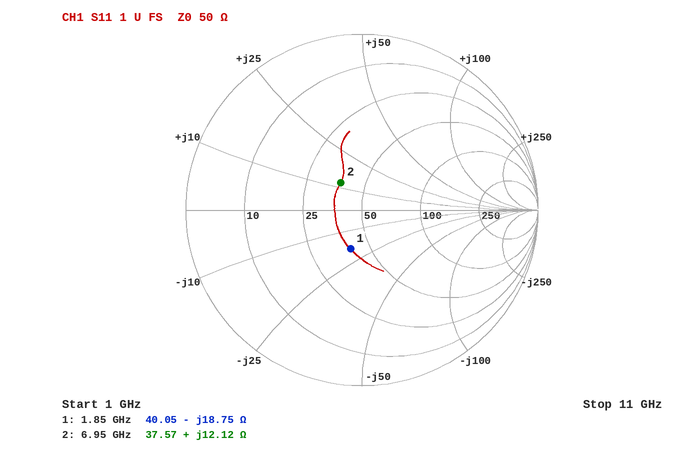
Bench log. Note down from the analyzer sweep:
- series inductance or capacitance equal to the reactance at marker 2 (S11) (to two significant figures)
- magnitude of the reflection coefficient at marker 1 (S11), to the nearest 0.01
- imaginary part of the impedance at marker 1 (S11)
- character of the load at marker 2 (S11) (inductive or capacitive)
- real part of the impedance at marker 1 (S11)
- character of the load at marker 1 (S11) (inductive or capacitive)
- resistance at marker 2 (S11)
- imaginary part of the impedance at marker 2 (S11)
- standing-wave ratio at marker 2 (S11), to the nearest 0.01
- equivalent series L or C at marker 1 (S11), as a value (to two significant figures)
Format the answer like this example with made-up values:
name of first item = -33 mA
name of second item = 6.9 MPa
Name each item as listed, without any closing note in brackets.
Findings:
series inductance or capacitance equal to the reactance at marker 2 (S11) = 280 pH
magnitude of the reflection coefficient at marker 1 (S11), to the nearest 0.01 = 0.23
imaginary part of the impedance at marker 1 = -18.75 Ω
character of the load at marker 2 (S11) = inductive
real part of the impedance at marker 1 = 40.05 Ω
character of the load at marker 1 (S11) = capacitive
resistance at marker 2 = 37.57 Ω
imaginary part of the impedance at marker 2 = +12.12 Ω
standing-wave ratio at marker 2 (S11), to the nearest 0.01 = 1.49
equivalent series L or C at marker 1 (S11), as a value = 4.6 pF
